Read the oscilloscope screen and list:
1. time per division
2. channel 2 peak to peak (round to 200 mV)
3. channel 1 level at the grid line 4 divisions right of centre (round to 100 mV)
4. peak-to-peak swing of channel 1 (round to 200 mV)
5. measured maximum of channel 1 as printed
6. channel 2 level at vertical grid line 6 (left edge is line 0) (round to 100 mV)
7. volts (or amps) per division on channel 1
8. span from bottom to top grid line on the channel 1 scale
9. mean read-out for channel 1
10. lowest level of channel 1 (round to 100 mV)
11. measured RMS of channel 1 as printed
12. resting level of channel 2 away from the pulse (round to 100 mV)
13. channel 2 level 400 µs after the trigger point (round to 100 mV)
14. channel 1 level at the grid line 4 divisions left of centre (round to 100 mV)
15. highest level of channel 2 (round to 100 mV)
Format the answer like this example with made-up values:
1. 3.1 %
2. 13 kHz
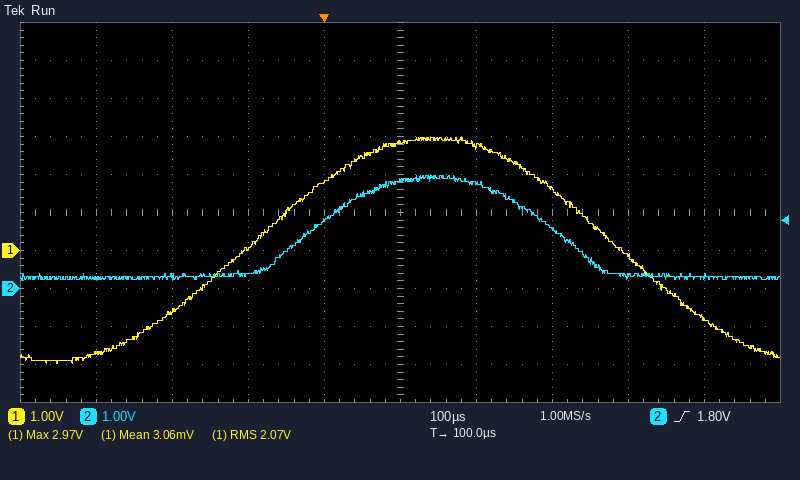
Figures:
1. 100 µs
2. 2.8 V
3. -1.8 V
4. 6.0 V
5. 2.97 V
6. 2.8 V
7. 1 V
8. 10 V
9. 3.06 mV
10. -3.0 V
11. 2.07 V
12. 300 mV
13. 300 mV
14. -2.7 V
15. 3.0 V
